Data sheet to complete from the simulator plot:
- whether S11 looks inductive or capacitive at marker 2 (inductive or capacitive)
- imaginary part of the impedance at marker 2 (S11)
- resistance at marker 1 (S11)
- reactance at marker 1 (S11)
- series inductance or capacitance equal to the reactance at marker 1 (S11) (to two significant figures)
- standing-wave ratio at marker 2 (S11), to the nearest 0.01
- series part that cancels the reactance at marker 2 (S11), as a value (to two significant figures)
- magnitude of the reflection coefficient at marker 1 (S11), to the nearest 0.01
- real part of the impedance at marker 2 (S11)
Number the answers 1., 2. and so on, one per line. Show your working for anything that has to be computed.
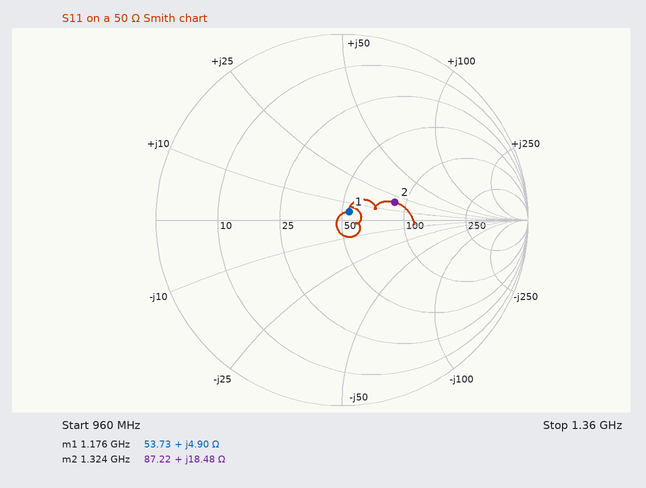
1. inductive
2. +18.48 Ω
3. 53.73 Ω
4. +4.90 Ω
5. L = 4.9 Ω/(2π × 1.176 GHz) ≈ 663 pH, so 660 pH to two significant figures
6. 1.86
7. C = 1/(2π × 1.324 GHz × 18.48 Ω) ≈ 6.5 pF
8. 0.06
9. 87.22 Ω
